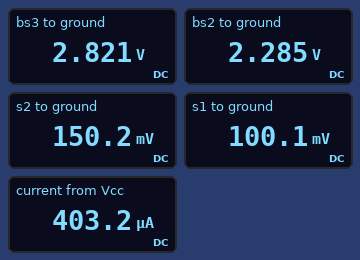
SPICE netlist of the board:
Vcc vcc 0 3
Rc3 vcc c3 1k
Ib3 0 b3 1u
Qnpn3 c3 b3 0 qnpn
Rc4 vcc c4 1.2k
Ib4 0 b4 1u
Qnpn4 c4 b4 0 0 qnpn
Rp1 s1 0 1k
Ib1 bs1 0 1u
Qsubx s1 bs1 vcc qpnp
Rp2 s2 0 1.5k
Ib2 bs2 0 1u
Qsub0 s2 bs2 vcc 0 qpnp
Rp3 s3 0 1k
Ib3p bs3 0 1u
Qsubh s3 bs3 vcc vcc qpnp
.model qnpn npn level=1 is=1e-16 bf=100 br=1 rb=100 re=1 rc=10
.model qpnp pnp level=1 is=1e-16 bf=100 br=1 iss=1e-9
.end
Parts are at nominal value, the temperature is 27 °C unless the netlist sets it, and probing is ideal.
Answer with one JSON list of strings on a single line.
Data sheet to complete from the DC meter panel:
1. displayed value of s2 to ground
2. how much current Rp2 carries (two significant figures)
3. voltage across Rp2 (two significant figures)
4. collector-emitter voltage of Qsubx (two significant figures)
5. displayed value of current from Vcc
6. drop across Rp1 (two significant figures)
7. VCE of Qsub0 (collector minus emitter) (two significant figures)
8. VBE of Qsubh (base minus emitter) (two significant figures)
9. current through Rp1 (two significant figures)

["150.2 mV", "100 µA", "150 mV", "-2.9 V", "403.2 µA", "100 mV", "-2.8 V", "-180 mV", "100 µA"]
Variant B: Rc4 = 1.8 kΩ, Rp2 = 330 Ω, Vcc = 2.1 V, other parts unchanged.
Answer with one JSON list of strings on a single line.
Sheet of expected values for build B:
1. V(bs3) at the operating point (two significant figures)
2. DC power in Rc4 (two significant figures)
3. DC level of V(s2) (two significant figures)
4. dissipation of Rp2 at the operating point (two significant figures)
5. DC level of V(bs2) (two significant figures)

["1.9 V", "18 µW", "33 mV", "3.3 µW", "1.4 V"]
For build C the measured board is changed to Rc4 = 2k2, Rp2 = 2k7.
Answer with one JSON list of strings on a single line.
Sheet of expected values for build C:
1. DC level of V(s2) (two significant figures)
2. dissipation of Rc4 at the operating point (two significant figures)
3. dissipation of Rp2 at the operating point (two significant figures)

["270 mV", "22 µW", "27 µW"]
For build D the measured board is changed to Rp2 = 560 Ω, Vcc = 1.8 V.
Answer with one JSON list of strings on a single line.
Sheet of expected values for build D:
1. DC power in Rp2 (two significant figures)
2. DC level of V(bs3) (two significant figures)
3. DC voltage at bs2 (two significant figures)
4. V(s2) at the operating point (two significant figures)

["5.6 µW", "1.6 V", "1.1 V", "56 mV"]
